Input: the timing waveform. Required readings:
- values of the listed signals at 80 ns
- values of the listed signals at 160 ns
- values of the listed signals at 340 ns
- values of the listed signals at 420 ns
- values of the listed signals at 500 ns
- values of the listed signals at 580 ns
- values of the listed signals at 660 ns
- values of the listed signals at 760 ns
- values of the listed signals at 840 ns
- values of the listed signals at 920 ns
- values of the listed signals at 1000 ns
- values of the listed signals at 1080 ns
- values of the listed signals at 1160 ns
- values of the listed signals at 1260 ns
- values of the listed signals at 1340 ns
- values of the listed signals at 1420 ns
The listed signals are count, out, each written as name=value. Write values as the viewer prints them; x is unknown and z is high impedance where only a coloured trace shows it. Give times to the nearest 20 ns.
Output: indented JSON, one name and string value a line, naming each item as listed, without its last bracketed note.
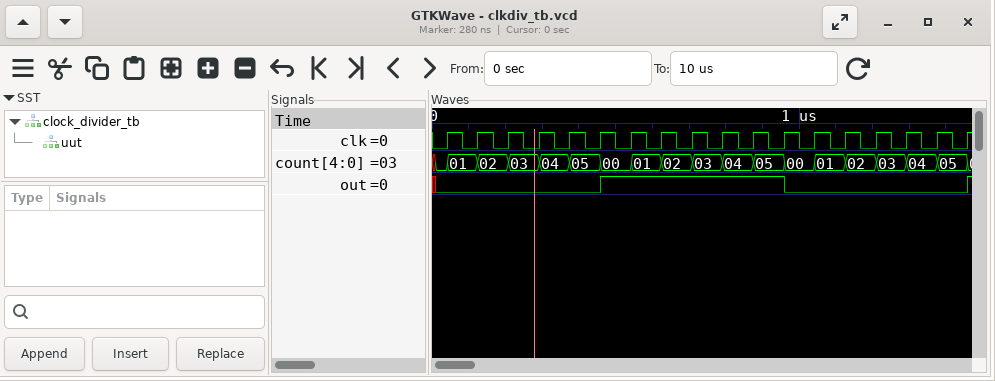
{
  "values of the listed signals at 80 ns": "count=01, out=0",
  "values of the listed signals at 160 ns": "count=02, out=0",
  "values of the listed signals at 340 ns": "count=04, out=0",
  "values of the listed signals at 420 ns": "count=05, out=0",
  "values of the listed signals at 500 ns": "count=00, out=1",
  "values of the listed signals at 580 ns": "count=01, out=1",
  "values of the listed signals at 660 ns": "count=02, out=1",
  "values of the listed signals at 760 ns": "count=03, out=1",
  "values of the listed signals at 840 ns": "count=04, out=1",
  "values of the listed signals at 920 ns": "count=05, out=1",
  "values of the listed signals at 1000 ns": "count=00, out=0",
  "values of the listed signals at 1080 ns": "count=01, out=0",
  "values of the listed signals at 1160 ns": "count=02, out=0",
  "values of the listed signals at 1260 ns": "count=03, out=0",
  "values of the listed signals at 1340 ns": "count=04, out=0",
  "values of the listed signals at 1420 ns": "count=05, out=0"
}
